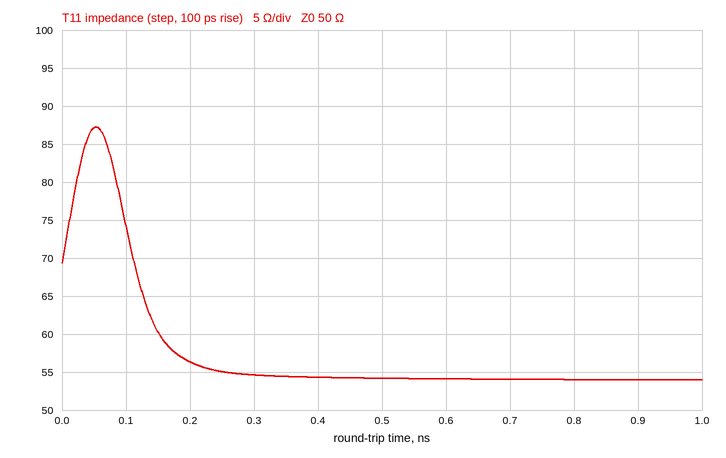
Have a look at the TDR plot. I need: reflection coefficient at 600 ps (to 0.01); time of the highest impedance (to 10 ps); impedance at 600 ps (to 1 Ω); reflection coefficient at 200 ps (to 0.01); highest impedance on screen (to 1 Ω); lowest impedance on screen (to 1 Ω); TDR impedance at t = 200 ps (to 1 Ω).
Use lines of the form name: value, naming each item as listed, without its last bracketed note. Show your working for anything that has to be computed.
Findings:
reflection coefficient at 600 ps: (54 − 50)/(54 + 50) ≈ +0.04
time of the highest impedance: 50 ps
impedance at 600 ps: 54 Ω
reflection coefficient at 200 ps: (56 − 50)/(56 + 50) ≈ +0.06
highest impedance on screen: 87 Ω
lowest impedance on screen: 54 Ω
TDR impedance at t = 200 ps: 56 Ω
